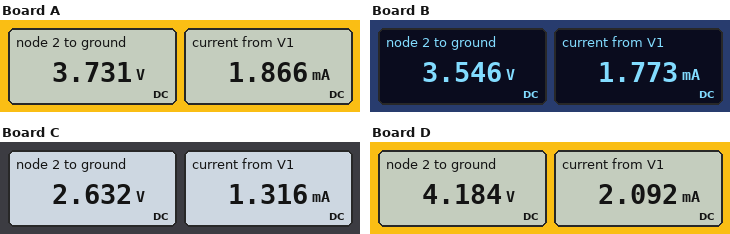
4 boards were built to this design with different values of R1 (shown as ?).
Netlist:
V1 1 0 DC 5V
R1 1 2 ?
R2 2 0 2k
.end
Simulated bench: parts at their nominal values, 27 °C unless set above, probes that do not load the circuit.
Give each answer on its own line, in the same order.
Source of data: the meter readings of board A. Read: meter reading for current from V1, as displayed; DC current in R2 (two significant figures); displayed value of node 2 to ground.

1.866 mA
1.9 mA
3.731 V
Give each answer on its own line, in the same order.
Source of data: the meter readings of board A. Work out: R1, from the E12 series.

680 Ω
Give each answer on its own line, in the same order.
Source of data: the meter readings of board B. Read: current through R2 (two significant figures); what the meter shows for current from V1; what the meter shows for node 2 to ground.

1.8 mA
1.773 mA
3.546 V
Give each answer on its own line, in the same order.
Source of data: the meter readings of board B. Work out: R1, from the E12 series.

820 Ω
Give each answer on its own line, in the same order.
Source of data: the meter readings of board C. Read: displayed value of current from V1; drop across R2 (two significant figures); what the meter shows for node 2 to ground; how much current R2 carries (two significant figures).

1.316 mA
2.6 V
2.632 V
1.3 mA
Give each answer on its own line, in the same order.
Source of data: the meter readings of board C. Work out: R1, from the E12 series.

1.8 kΩ
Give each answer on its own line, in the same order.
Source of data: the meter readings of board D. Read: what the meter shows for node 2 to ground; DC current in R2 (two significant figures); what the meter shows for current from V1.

4.184 V
2.1 mA
2.092 mA
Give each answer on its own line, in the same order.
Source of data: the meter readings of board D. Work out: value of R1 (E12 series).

390 Ω
